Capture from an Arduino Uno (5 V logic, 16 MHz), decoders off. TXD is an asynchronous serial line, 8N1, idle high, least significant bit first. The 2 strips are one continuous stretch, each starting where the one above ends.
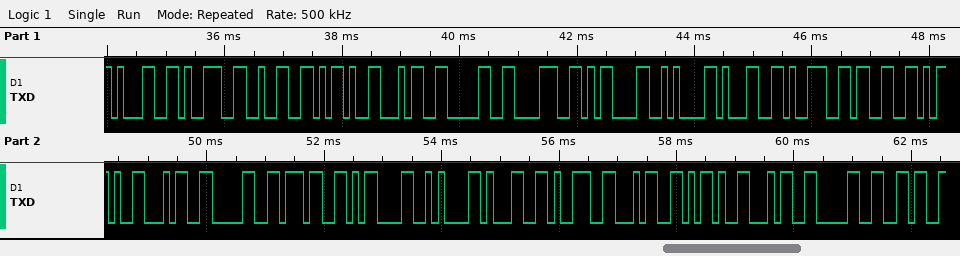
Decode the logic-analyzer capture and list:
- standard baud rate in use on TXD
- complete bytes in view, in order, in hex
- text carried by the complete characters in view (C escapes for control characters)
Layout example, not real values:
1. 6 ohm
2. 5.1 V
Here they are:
1. 9600 baud
2. 31 39 32 2D 34 30 38 0D 0A 31 39 33 2D 34 30 37 0D 0A 31 39 34 2D 34 30 36
3. "192-408\r\n193-407\r\n194-406"
